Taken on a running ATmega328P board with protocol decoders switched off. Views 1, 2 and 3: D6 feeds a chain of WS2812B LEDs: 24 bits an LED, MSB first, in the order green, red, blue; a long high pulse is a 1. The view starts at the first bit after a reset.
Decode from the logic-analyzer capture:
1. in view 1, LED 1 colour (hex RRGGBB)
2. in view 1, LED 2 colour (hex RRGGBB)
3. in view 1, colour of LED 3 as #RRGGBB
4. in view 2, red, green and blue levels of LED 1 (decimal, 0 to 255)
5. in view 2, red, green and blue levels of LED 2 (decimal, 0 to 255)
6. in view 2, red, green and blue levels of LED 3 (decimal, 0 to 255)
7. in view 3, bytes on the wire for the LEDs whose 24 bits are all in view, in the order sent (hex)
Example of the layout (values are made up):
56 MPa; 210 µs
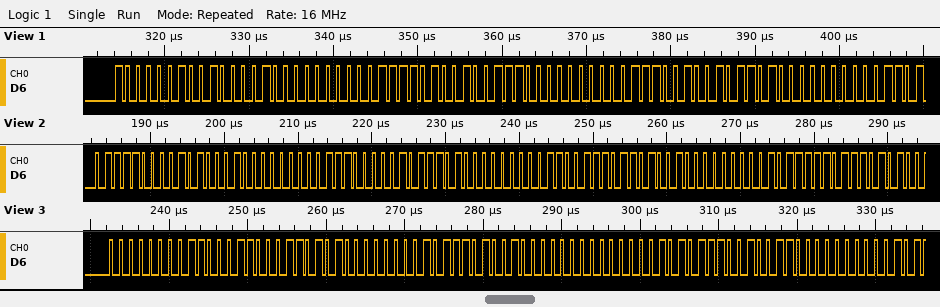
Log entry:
#428200; #4E7A00; #5A7200; 81, 120, 0; 93, 112, 0; 105, 103, 0; 00 C6 35 00 BA 40 00 AE 4C
